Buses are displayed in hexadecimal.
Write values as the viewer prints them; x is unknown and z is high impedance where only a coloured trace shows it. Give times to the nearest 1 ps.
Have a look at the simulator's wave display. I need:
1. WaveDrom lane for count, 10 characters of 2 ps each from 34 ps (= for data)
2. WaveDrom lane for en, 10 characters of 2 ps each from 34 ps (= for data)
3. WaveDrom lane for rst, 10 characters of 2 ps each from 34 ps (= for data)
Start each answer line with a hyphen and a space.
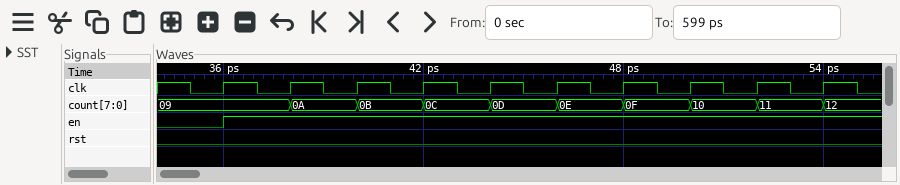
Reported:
- {name: 'count', wave: '=.========', data: '09 0A 0B 0C 0D 0E 0F 10 11'}
- {name: 'en', wave: '01........'}
- {name: 'rst', wave: '0.........'}
